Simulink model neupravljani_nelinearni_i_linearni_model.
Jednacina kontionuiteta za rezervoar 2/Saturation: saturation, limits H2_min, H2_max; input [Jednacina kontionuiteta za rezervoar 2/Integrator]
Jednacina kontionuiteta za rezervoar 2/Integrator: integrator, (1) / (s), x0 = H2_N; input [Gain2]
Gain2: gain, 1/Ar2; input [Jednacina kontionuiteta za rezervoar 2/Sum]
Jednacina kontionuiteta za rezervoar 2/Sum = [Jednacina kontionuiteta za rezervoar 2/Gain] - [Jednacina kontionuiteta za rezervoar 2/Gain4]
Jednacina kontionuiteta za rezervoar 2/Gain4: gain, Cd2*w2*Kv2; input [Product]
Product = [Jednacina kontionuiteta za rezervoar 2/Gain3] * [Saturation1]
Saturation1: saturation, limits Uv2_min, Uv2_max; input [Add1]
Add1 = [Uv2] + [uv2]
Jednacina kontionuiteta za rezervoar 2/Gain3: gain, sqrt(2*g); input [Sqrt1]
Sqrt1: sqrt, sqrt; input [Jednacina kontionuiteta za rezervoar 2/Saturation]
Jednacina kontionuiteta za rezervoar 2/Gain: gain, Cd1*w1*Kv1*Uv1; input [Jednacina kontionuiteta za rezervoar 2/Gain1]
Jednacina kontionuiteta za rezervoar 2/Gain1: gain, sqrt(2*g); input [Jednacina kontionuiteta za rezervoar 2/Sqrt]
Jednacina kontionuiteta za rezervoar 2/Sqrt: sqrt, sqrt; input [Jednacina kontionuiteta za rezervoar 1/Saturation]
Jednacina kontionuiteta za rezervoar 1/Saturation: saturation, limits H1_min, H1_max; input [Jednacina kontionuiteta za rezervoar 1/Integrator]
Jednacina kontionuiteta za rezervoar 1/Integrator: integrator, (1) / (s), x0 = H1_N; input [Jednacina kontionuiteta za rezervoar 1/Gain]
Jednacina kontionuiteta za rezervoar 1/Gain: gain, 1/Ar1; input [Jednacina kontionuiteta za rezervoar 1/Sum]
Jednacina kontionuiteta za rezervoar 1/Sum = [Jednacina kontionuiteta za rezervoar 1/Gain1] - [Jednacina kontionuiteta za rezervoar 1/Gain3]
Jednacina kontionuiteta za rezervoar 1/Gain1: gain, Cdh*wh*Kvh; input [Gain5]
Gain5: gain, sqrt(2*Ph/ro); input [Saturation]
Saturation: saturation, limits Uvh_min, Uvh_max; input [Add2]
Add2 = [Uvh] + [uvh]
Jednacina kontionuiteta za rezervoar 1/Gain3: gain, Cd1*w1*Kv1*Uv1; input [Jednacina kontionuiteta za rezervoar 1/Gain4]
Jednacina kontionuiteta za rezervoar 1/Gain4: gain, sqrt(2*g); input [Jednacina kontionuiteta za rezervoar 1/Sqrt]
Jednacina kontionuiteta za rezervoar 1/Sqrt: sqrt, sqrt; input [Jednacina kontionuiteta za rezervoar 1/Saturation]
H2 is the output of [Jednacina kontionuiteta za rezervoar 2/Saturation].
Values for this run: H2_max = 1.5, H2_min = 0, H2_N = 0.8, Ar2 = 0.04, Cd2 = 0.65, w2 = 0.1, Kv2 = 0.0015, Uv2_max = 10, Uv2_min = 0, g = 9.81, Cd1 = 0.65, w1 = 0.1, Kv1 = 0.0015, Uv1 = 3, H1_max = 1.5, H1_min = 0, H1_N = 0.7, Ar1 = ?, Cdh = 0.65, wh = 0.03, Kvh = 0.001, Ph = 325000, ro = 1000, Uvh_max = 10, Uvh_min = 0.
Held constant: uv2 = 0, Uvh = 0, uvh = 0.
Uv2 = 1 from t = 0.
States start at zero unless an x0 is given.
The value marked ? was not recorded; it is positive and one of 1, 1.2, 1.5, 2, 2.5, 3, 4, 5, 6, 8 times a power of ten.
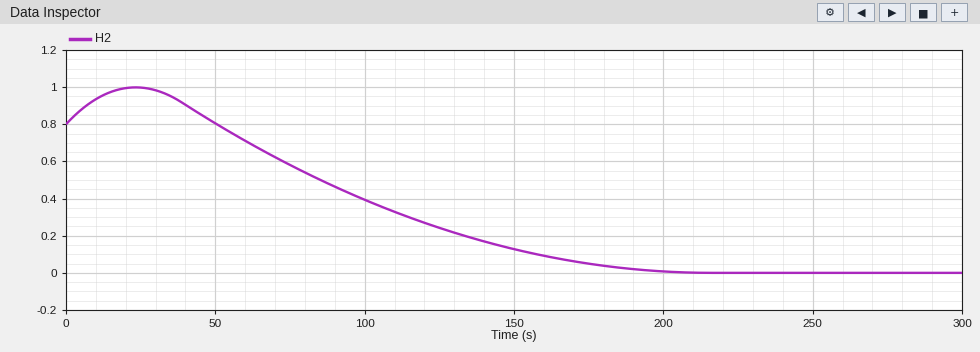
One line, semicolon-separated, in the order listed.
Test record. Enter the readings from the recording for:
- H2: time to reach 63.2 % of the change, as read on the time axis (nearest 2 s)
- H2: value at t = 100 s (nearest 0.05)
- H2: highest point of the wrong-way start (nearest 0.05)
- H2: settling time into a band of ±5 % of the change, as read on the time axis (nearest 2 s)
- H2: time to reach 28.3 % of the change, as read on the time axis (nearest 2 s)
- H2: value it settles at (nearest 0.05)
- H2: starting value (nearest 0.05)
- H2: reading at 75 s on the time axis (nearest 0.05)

116 s; 0.40; 1.00; 180 s; 76 s; 0.00; 0.80; 0.60
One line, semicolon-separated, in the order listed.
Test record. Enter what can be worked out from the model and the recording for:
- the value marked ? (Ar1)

0.03
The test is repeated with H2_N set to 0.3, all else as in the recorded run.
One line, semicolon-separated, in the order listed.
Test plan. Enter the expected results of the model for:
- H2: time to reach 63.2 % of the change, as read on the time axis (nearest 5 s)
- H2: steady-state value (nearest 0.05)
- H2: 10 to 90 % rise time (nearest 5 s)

110 s; 0.00; 65 s
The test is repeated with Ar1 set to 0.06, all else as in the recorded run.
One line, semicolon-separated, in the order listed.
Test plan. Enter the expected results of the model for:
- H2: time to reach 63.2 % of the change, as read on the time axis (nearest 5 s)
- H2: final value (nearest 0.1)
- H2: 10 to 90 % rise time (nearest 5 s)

160 s; 0.0; 105 s
